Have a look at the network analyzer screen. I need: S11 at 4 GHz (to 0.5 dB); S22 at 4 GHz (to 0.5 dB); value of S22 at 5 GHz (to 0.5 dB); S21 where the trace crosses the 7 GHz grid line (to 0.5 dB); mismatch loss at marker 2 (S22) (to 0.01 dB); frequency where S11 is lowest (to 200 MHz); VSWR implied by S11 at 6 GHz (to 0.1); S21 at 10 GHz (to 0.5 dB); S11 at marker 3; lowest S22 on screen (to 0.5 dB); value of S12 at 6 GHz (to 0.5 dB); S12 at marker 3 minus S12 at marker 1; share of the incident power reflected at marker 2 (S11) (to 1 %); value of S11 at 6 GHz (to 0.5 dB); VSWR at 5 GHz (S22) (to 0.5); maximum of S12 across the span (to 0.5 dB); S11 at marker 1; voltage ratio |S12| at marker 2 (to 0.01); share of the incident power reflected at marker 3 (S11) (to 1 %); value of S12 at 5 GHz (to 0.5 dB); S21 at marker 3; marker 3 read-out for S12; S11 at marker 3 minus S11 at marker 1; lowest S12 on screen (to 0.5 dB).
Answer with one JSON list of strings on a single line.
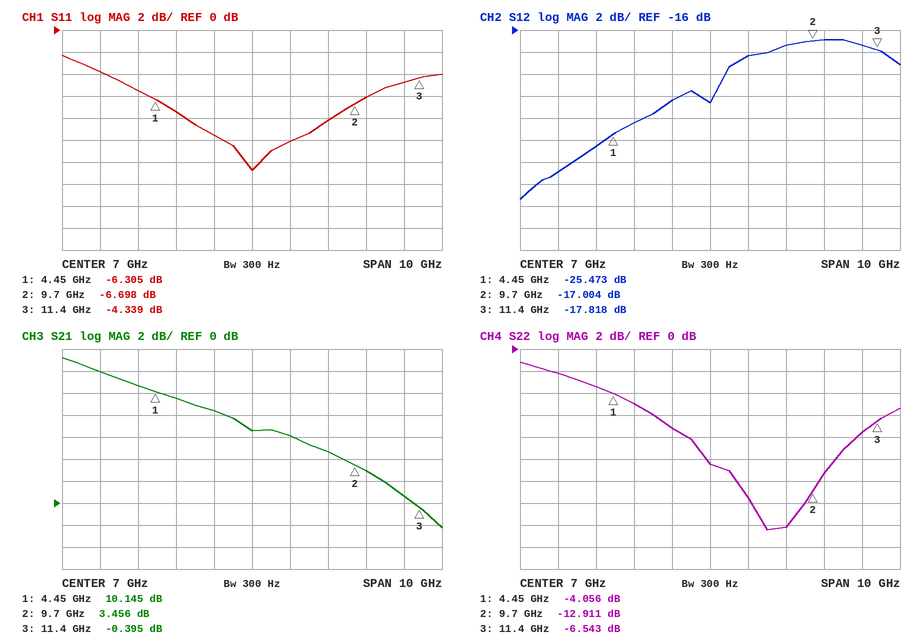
["-5.5 dB", "-3.5 dB", "-5.0 dB", "6.5 dB", "0.23 dB", "7.0 GHz", "2.0", "3.0 dB", "-4.339 dB", "-16.5 dB", "-22.5 dB", "7.655 dB", "21 %", "-9.5 dB", "3.5", "-17.0 dB", "-6.305 dB", "0.14", "37 %", "-24.5 dB", "-0.395 dB", "-17.818 dB", "1.966 dB", "-31.5 dB"]
